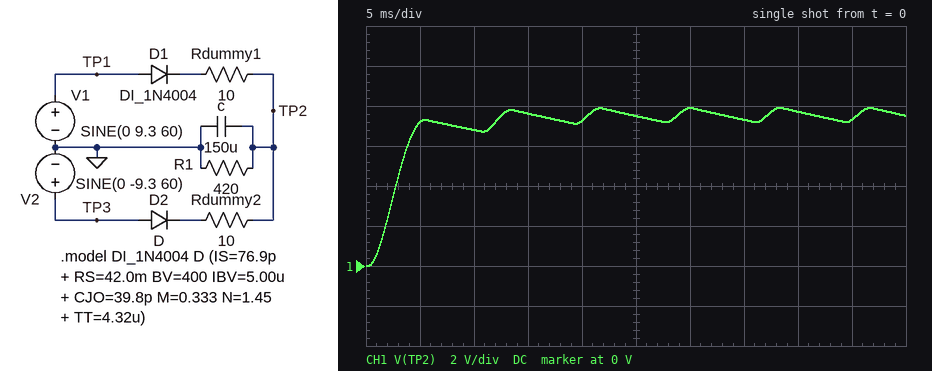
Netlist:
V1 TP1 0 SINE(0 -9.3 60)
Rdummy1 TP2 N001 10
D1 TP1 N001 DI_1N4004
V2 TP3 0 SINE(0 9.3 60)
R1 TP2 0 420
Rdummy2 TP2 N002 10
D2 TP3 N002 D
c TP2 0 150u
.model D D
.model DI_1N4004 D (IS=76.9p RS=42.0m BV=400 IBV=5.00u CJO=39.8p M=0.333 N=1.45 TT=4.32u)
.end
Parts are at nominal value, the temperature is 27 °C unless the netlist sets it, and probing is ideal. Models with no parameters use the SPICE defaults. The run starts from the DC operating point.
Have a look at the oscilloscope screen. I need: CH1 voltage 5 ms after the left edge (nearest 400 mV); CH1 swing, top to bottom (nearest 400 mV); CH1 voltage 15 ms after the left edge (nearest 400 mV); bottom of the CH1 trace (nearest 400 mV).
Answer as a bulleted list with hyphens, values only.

- 7.2 V
- 8.0 V
- 7.6 V
- 0 V
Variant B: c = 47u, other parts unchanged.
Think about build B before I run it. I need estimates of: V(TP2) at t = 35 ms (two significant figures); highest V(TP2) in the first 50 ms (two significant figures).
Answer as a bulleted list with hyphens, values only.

- 6.3 V
- 8.2 V
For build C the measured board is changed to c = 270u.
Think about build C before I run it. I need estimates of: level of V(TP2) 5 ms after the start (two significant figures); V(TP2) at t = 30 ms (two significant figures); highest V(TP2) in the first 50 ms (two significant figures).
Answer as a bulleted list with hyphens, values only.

- 5.8 V
- 7.7 V
- 7.8 V
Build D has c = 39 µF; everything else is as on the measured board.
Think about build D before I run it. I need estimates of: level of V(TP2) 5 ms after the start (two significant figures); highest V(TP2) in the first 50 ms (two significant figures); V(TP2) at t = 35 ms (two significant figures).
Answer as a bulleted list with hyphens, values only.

- 8.2 V
- 8.3 V
- 6.0 V
